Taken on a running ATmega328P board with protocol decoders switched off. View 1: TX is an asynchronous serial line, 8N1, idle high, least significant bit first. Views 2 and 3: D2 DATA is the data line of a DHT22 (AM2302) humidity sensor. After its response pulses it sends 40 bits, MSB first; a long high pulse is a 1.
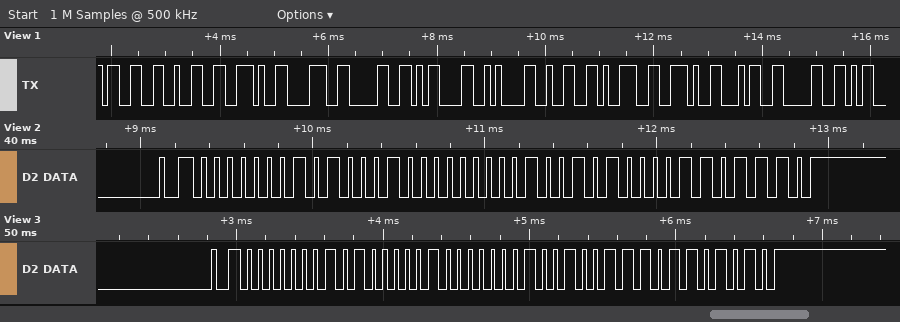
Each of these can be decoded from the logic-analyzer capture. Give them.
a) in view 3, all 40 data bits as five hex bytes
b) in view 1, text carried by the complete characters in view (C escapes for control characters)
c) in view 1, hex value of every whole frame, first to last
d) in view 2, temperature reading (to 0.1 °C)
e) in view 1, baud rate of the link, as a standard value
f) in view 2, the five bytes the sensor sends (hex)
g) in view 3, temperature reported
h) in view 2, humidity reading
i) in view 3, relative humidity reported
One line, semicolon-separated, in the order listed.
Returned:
01 41 01 27 6A; "32.80\r\n29.40"; 33 32 2E 38 30 0D 0A 32 39 2E 34 30; 29.6 °C; 9600 baud; 01 44 01 28 6E; 29.5 °C; 32.4 %; 32.1 %
